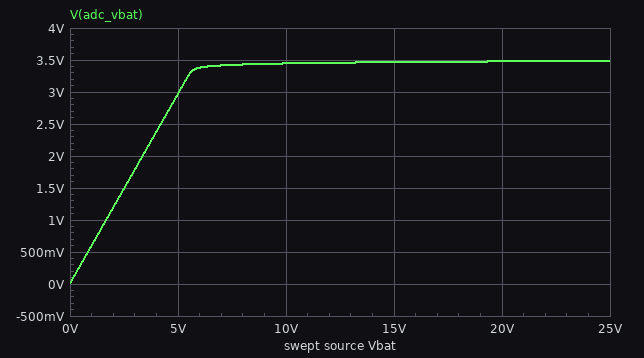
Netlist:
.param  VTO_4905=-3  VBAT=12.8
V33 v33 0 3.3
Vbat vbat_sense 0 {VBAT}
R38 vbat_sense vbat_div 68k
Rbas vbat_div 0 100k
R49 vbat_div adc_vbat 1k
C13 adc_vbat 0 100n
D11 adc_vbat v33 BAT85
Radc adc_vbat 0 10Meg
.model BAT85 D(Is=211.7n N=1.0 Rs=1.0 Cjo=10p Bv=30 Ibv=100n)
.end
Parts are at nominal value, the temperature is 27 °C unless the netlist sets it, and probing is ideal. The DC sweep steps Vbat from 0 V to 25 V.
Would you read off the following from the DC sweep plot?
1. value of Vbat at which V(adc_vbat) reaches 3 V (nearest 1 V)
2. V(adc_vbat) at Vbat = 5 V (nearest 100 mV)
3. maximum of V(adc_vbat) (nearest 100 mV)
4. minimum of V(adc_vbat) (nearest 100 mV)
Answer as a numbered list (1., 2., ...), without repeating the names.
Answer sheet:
1. 5 V
2. 3.0 V
3. 3.5 V
4. 0 V
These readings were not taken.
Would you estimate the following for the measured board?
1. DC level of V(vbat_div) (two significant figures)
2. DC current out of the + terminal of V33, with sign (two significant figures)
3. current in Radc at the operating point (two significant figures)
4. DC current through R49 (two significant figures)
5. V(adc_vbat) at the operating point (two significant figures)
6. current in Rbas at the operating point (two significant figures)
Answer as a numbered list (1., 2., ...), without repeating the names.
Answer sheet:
1. 3.6 V
2. -100 µA
3. 350 nA
4. 100 µA
5. 3.5 V
6. 36 µA
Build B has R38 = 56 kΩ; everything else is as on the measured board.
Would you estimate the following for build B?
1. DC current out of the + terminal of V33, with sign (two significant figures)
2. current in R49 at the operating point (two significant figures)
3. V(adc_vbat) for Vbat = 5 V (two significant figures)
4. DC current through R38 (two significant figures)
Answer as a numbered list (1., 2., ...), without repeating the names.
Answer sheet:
1. -130 µA
2. 130 µA
3. 3.2 V
4. 160 µA
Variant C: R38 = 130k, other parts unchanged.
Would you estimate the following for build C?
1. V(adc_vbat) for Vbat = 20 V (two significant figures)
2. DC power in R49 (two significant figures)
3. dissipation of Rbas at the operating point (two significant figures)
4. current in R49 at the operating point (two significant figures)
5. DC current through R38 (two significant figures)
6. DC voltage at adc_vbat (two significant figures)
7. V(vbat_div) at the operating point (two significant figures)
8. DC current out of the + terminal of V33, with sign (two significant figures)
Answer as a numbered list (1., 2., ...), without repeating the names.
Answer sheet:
1. 3.5 V
2. 1.4 µW
3. 120 µW
4. 37 µA
5. 72 µA
6. 3.4 V
7. 3.5 V
8. -37 µA
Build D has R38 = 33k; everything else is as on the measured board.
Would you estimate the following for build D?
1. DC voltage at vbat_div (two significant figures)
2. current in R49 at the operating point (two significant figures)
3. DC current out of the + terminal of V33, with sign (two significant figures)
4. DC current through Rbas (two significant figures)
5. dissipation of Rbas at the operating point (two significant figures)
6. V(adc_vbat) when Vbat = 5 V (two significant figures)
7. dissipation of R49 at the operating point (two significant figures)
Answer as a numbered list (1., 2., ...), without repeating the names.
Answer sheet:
1. 3.7 V
2. 240 µA
3. -240 µA
4. 37 µA
5. 140 µW
6. 3.4 V
7. 57 µW
